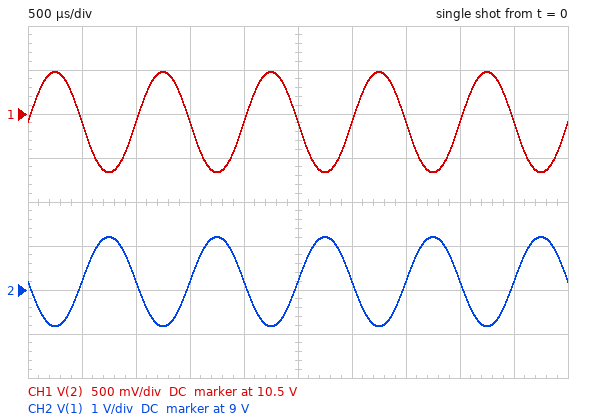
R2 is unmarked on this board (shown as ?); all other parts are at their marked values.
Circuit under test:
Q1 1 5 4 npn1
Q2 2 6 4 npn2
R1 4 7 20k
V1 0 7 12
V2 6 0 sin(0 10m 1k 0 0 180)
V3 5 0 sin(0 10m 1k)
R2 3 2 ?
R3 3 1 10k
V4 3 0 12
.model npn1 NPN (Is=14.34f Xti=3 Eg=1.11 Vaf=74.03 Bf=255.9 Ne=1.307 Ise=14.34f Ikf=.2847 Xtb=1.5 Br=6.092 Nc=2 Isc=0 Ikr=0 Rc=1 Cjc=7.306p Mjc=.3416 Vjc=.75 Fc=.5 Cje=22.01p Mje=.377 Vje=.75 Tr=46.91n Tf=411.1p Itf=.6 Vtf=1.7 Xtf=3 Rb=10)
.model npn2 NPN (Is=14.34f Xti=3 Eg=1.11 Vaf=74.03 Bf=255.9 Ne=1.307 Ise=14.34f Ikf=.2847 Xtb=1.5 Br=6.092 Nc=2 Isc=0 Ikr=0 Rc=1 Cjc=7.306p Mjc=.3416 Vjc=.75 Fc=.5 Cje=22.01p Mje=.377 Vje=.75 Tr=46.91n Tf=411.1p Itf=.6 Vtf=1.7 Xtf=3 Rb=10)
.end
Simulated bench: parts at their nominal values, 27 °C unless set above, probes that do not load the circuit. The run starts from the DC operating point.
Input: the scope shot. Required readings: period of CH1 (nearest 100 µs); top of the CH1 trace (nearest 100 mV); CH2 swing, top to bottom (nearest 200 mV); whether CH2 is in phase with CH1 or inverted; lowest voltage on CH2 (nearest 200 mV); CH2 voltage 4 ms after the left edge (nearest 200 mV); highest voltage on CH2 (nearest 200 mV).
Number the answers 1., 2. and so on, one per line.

1. 1.0 ms
2. 11.0 V
3. 2.0 V
4. inverted
5. 8.2 V
6. 9.2 V
7. 10.2 V
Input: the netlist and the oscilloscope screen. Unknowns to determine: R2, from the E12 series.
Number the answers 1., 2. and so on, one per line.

1. 5.6 kΩ
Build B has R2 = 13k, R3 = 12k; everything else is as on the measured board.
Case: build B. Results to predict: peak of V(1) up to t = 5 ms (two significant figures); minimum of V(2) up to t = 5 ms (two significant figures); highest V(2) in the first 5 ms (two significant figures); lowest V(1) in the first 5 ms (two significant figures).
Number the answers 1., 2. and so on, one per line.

1. 9.8 V
2. 7.0 V
3. 9.6 V
4. 7.4 V
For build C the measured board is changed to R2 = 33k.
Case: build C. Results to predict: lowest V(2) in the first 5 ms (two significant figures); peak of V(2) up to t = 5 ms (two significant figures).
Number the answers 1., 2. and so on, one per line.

1. -220 mV
2. 6.2 V
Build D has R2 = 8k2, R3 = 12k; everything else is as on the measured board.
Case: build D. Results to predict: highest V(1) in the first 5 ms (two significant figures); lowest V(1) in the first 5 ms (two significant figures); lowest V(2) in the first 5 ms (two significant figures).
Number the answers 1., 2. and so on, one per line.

1. 9.8 V
2. 7.4 V
3. 8.8 V
